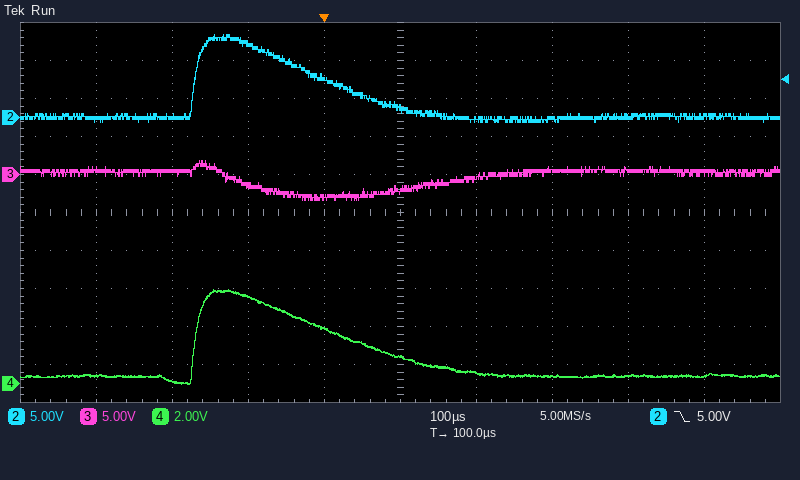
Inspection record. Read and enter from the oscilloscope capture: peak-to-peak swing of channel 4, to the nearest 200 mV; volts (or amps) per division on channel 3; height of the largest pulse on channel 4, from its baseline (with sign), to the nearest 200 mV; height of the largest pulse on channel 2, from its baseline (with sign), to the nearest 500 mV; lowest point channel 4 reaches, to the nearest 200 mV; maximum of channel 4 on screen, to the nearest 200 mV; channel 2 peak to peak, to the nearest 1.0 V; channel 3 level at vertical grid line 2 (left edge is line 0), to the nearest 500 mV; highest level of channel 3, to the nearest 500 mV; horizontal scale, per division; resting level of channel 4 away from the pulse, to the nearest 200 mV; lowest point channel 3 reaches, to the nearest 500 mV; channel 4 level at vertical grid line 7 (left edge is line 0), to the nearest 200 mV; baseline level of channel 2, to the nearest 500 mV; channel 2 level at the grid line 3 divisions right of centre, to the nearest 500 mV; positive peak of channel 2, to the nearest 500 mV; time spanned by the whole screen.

5.0 V
5 V
+4.6 V
+11.0 V
0.0 V
5.0 V
12.0 V
500 mV
2.0 V
100 µs
400 mV
-3.5 V
400 mV
0.0 V
0.0 V
11.0 V
1 ms
